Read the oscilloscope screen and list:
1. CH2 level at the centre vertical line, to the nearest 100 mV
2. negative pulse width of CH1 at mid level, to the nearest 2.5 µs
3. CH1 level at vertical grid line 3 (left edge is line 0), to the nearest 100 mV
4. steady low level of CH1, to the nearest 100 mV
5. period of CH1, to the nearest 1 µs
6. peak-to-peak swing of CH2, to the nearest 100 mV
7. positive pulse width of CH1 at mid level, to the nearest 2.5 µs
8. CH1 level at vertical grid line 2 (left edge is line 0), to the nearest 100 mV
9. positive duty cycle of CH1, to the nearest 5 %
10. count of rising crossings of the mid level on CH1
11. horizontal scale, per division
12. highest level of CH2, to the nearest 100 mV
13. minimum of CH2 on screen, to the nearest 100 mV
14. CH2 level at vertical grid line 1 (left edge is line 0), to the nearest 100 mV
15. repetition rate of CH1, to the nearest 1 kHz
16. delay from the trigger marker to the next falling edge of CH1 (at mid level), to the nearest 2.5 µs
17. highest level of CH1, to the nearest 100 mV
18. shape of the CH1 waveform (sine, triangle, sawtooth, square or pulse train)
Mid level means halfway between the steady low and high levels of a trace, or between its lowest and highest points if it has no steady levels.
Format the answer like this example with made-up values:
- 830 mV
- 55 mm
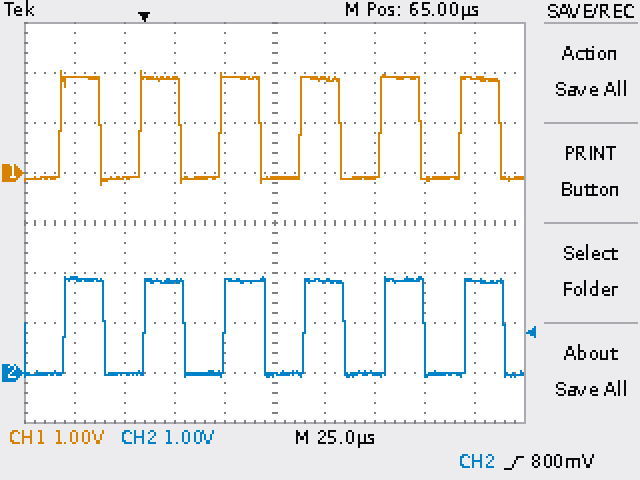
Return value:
- 0.0 V
- 20.0 µs
- 1.9 V
- -100 mV
- 40 µs
- 2.0 V
- 20.0 µs
- -100 mV
- 50 %
- 6
- 25 µs
- 1.9 V
- -100 mV
- 1.9 V
- 25 kHz
- 17.5 µs
- 2.0 V
- square
